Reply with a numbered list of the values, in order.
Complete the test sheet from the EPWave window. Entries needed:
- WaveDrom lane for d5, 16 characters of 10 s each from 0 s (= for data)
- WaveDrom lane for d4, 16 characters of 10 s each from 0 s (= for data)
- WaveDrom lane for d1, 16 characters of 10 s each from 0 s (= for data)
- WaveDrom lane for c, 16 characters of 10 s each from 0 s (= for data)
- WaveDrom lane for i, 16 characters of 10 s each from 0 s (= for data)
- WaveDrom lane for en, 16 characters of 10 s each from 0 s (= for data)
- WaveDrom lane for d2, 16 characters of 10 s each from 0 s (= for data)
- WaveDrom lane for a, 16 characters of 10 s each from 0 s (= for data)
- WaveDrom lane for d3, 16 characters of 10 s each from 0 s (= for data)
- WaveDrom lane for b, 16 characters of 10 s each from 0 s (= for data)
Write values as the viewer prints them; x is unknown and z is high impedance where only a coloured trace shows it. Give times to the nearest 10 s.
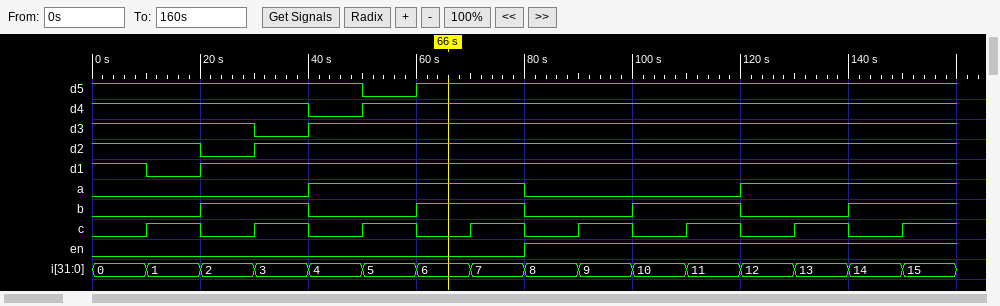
1. {name: 'd5', wave: '1....01.........'}
2. {name: 'd4', wave: '1...01..........'}
3. {name: 'd1', wave: '101.............'}
4. {name: 'c', wave: '0101010101010101'}
5. {name: 'i', wave: '================', data: '0 1 2 3 4 5 6 7 8 9 10 11 12 13 14 15'}
6. {name: 'en', wave: '0.......1.......'}
7. {name: 'd2', wave: '1.01............'}
8. {name: 'a', wave: '0...1...0...1...'}
9. {name: 'd3', wave: '1..01...........'}
10. {name: 'b', wave: '0.1.0.1.0.1.0.1.'}
